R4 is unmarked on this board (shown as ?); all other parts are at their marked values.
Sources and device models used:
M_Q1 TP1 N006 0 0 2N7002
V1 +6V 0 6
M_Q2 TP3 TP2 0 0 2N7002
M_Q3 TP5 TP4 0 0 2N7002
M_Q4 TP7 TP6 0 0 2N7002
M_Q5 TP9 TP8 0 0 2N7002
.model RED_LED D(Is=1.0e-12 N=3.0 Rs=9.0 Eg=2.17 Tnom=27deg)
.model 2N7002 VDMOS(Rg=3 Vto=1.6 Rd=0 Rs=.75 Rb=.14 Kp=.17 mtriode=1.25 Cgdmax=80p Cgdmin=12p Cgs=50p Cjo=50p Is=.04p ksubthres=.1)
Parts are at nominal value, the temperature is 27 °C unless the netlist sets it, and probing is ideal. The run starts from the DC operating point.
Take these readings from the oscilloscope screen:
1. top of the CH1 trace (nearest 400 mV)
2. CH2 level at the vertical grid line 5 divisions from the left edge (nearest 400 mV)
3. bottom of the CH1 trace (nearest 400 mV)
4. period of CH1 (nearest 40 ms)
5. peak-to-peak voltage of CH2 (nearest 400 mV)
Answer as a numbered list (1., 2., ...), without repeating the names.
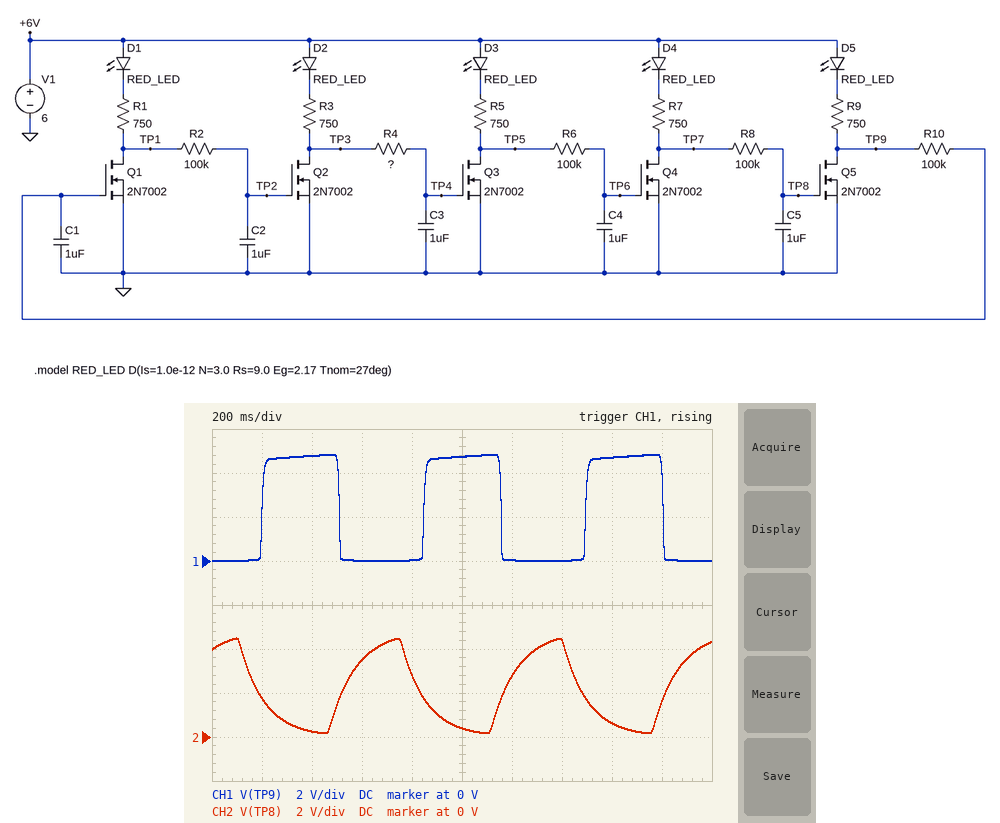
1. 4.8 V
2. 400 mV
3. 0 V
4. 640 ms
5. 4.4 V
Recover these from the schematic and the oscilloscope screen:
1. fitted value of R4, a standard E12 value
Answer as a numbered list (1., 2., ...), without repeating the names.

1. 56 kΩ
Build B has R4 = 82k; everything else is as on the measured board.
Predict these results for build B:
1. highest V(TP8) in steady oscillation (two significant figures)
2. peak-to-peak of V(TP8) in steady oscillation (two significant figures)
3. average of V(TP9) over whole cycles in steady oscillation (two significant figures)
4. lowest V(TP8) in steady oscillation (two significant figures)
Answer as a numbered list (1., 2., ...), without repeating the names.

1. 4.6 V
2. 4.4 V
3. 2.2 V
4. 140 mV
